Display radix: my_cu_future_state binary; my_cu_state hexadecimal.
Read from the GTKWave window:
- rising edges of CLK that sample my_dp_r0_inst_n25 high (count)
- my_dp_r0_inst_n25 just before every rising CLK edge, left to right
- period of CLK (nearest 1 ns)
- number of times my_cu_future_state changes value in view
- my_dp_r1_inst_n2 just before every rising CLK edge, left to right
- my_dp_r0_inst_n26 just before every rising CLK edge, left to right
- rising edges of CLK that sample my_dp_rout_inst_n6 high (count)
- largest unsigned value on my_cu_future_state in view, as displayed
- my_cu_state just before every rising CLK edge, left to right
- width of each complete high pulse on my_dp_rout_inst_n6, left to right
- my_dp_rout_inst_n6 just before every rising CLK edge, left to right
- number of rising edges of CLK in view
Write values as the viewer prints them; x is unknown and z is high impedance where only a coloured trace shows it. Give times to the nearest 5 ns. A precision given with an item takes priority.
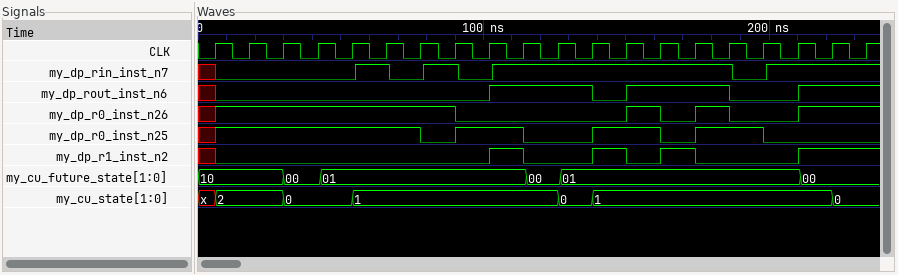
12
x 1 1 1 1 1 1 0 1 1 0 0 1 1 0 1 1 0 0 0
12 ns
5
x 0 0 0 0 0 0 0 0 1 0 0 1 0 1 0 0 0 1 1
x 1 1 1 1 1 1 1 0 0 0 0 0 1 0 1 0 0 1 1
8
10
x, 2, 2, 0, 0, 1, 1, 1, 1, 1, 1, 0, 1, 1, 1, 1, 1, 1, 1, 0
35 ns, 35 ns
x 0 0 0 0 0 0 0 0 1 1 1 0 1 1 1 0 0 1 1
20
